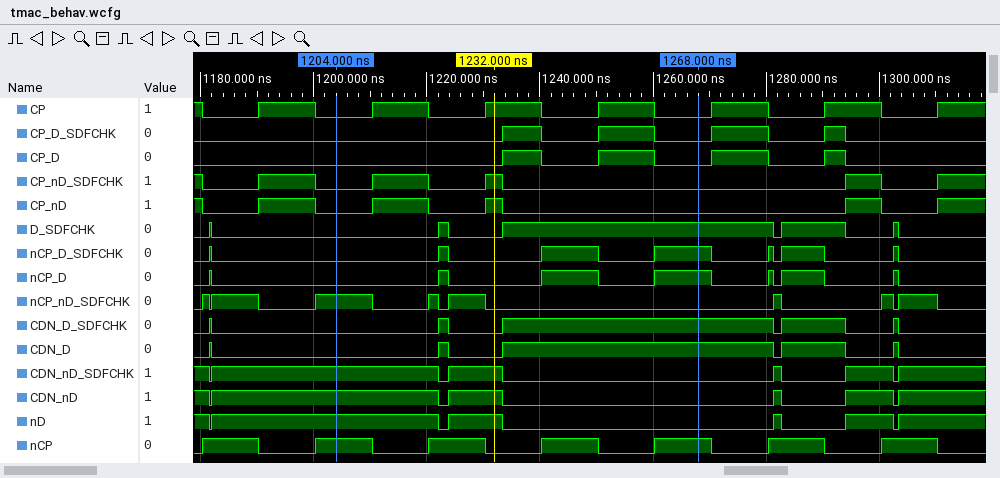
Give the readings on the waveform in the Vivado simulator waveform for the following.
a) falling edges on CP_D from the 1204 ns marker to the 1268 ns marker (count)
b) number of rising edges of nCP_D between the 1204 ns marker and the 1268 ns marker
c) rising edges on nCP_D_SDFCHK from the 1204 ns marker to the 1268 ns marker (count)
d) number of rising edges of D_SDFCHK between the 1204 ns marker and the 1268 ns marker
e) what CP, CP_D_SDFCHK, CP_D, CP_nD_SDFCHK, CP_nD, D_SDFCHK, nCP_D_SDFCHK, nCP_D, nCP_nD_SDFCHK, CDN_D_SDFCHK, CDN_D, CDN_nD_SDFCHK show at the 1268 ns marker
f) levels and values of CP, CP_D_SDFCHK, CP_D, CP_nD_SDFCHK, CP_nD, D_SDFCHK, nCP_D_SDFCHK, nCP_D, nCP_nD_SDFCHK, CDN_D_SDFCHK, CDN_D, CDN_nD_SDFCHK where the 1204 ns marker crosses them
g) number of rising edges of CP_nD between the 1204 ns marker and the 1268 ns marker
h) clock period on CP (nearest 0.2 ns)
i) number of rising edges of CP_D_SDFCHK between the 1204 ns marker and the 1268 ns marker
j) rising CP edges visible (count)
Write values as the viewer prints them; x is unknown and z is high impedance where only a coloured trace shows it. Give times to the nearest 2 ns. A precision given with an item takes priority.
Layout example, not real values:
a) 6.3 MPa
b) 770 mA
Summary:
a) 2
b) 3
c) 3
d) 2
e) CP=0, CP_D_SDFCHK=0, CP_D=0, CP_nD_SDFCHK=0, CP_nD=0, D_SDFCHK=1, nCP_D_SDFCHK=1, nCP_D=1, nCP_nD_SDFCHK=0, CDN_D_SDFCHK=1, CDN_D=1, CDN_nD_SDFCHK=0
f) CP=0, CP_D_SDFCHK=0, CP_D=0, CP_nD_SDFCHK=0, CP_nD=0, D_SDFCHK=0, nCP_D_SDFCHK=0, nCP_D=0, nCP_nD_SDFCHK=1, CDN_D_SDFCHK=0, CDN_D=0, CDN_nD_SDFCHK=1
g) 2
h) 20 ns
i) 2
j) 7
